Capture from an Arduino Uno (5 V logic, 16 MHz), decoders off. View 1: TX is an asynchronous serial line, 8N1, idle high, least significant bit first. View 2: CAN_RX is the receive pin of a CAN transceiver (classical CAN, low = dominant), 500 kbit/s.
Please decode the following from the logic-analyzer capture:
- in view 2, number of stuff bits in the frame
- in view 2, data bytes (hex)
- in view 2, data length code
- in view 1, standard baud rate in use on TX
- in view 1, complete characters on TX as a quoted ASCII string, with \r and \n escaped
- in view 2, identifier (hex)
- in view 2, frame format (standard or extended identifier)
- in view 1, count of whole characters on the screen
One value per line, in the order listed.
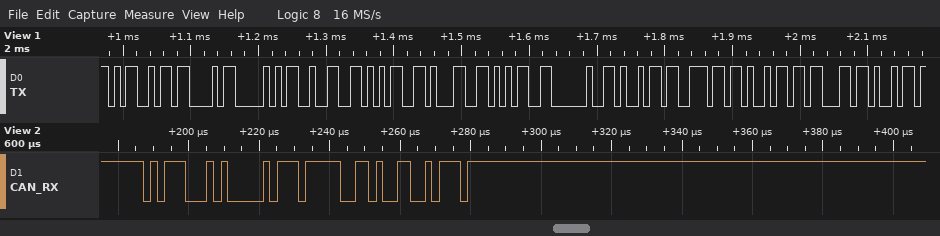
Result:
2
DF
1
115200 baud
"MCP2515 inici"
0x5C5
standard
13
